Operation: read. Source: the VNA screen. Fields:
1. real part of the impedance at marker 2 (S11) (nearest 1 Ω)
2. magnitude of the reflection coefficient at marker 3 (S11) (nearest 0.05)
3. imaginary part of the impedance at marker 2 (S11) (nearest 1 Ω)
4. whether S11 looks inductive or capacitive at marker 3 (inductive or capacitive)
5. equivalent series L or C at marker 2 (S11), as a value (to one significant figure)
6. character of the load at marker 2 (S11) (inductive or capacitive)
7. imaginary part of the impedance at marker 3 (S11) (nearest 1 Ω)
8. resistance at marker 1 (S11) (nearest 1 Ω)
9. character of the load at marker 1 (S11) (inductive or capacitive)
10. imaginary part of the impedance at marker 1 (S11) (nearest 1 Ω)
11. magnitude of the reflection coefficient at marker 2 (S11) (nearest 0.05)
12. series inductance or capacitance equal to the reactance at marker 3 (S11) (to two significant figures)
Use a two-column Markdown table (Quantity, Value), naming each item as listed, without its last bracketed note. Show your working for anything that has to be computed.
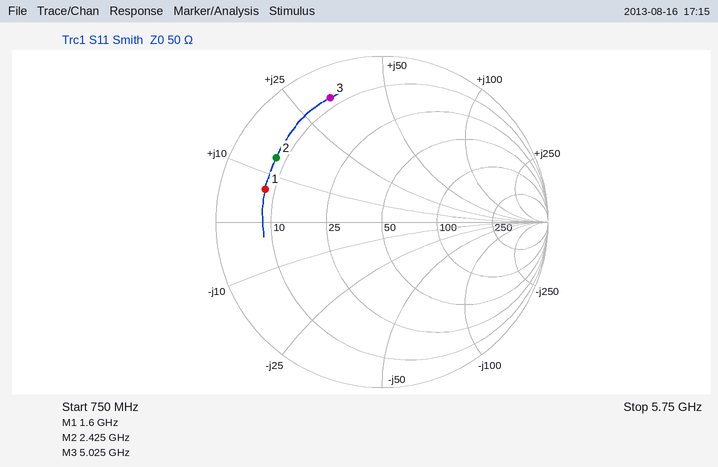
| Quantity | Value |
|---|---|
| real part of the impedance at marker 2 (S11) | 8 Ω |
| magnitude of the reflection coefficient at marker 3 (S11) | 0.80 |
| imaginary part of the impedance at marker 2 (S11) | +14 Ω |
| whether S11 looks inductive or capacitive at marker 3 | inductive |
| equivalent series L or C at marker 2 (S11), as a value | L = 14 Ω/(2π × 2.425 GHz) ≈ 919 pH, so 900 pH to one significant figure |
| character of the load at marker 2 (S11) | inductive |
| imaginary part of the impedance at marker 3 (S11) | +33 Ω |
| resistance at marker 1 (S11) | 8 Ω |
| character of the load at marker 1 (S11) | inductive |
| imaginary part of the impedance at marker 1 (S11) | +7 Ω |
| magnitude of the reflection coefficient at marker 2 (S11) | 0.75 |
| series inductance or capacitance equal to the reactance at marker 3 (S11) | L = 33 Ω/(2π × 5.025 GHz) ≈ 1.0 nH |
